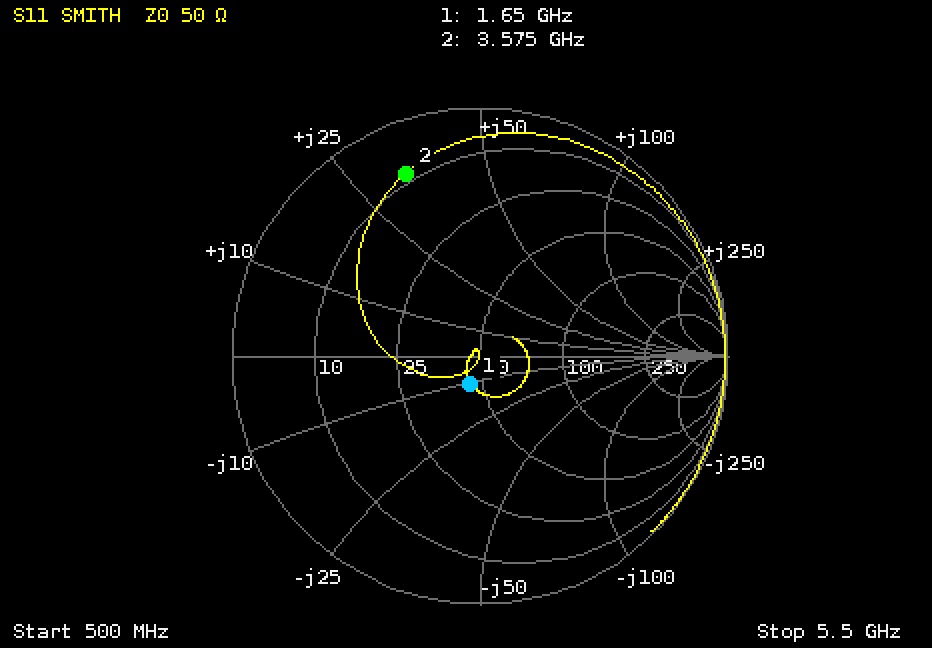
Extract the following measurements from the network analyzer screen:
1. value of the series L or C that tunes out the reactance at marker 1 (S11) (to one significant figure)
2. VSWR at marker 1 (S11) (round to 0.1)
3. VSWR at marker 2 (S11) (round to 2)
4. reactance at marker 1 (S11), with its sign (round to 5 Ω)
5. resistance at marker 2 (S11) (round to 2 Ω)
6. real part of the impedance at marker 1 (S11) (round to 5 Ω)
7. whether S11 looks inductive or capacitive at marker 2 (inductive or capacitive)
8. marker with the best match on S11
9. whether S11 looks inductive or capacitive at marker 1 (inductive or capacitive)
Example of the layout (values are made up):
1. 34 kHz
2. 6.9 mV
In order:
1. 1 nH
2. 1.3
3. 8
4. -10 Ω
5. 8 Ω
6. 45 Ω
7. inductive
8. marker 1
9. capacitive
